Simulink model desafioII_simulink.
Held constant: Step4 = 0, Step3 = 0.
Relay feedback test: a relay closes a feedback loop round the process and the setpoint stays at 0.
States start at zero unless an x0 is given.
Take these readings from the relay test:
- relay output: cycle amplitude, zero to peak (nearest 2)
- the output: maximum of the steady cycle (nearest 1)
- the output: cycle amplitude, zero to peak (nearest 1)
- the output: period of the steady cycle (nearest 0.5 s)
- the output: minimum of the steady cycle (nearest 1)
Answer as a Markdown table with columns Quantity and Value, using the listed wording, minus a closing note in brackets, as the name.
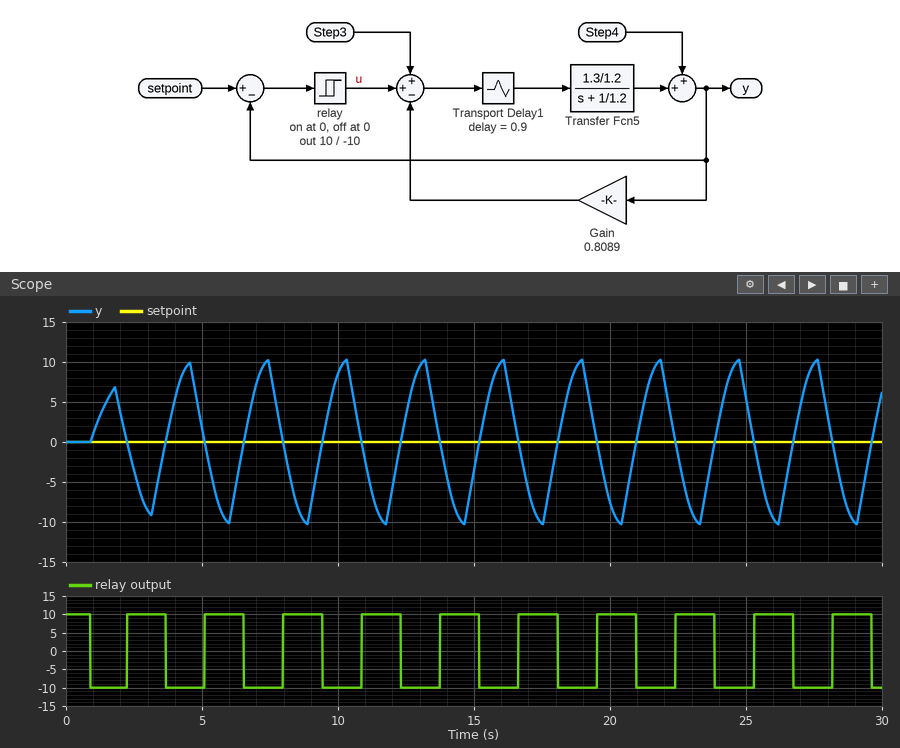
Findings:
| Quantity | Value |
|---|---|
| relay output: cycle amplitude, zero to peak | 10 |
| the output: maximum of the steady cycle | 10 |
| the output: cycle amplitude, zero to peak | 10 |
| the output: period of the steady cycle | 3.0 s |
| the output: minimum of the steady cycle | -10 |
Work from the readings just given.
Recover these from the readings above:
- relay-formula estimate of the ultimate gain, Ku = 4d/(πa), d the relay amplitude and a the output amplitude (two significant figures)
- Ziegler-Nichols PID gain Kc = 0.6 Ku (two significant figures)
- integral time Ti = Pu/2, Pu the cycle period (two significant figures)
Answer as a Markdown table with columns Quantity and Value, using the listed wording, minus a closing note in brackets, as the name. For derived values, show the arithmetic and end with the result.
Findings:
| Quantity | Value |
|---|---|
| relay-formula estimate of the ultimate gain, Ku = 4d/(πa), d the relay amplitude and a the output amplitude | 4 × 10 / (π × 10) = 1.3 |
| Ziegler-Nichols PID gain Kc = 0.6 Ku | 0.6 × 1.3 = 0.78 |
| integral time Ti = Pu/2, Pu the cycle period | 3 / 2 = 1.5 s |
